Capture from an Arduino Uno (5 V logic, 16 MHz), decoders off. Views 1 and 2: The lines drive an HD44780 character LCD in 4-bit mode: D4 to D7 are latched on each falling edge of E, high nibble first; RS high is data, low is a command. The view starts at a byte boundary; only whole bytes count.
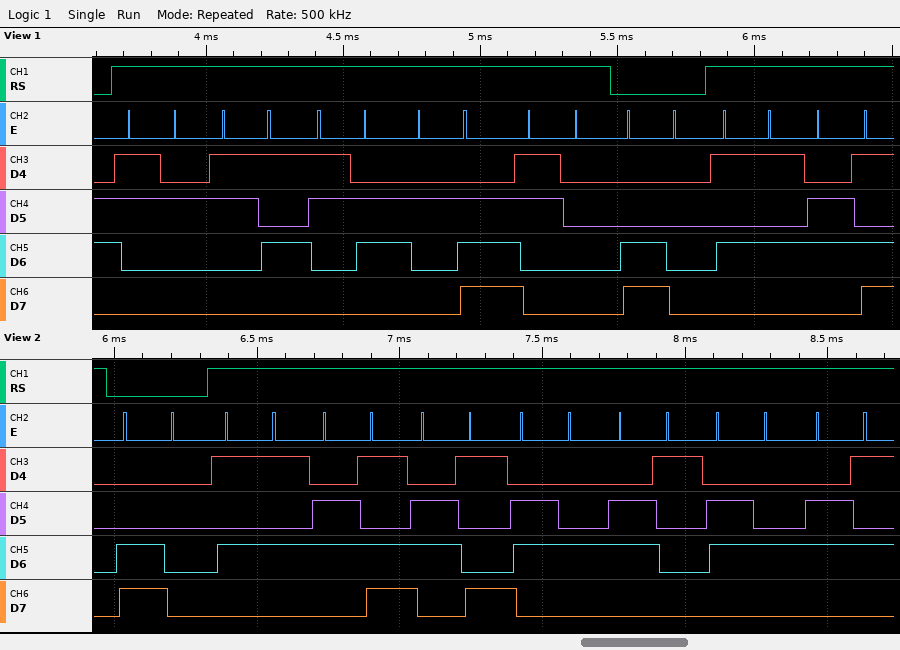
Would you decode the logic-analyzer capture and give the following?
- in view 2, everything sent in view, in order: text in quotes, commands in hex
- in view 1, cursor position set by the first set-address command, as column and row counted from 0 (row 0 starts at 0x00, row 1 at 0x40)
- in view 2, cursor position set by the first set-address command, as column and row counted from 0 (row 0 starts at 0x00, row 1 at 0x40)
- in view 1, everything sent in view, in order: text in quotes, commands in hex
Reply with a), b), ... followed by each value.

a) 0xC0 "Umidade"
b) column 0, row 1
c) column 0, row 1
d) "256.0" 0xC0 "Um"
